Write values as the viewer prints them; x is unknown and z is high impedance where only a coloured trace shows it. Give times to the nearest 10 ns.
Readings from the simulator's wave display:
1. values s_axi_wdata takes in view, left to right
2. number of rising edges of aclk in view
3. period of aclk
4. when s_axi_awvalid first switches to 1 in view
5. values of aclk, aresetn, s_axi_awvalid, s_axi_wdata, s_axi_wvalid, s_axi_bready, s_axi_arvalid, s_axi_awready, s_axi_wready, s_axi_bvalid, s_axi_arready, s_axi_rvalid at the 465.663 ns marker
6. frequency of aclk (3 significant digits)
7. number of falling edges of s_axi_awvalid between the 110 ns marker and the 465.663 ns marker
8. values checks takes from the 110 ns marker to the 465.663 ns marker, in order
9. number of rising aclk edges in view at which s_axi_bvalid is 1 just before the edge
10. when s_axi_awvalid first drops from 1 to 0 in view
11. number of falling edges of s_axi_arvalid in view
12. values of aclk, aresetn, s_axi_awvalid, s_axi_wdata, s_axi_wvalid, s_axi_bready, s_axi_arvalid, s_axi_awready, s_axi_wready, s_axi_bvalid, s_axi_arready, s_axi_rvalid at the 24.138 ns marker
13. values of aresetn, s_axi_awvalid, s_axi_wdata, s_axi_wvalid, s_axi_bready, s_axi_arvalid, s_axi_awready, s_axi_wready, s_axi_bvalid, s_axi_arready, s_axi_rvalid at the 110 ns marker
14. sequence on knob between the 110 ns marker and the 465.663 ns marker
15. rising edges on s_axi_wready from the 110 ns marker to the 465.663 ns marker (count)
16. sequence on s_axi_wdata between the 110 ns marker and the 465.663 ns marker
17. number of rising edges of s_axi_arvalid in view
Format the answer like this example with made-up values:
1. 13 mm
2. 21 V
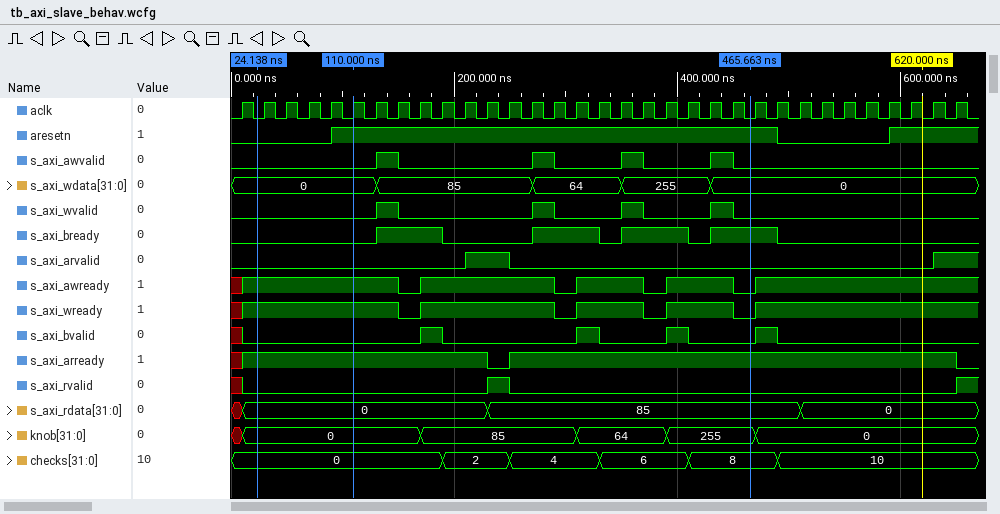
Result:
1. 0, 85, 64, 255, 0
2. 33
3. 20 ns
4. 130 ns
5. aclk=0, aresetn=1, s_axi_awvalid=0, s_axi_wdata=0, s_axi_wvalid=0, s_axi_bready=1, s_axi_arvalid=0, s_axi_awready=0, s_axi_wready=0, s_axi_bvalid=0, s_axi_arready=1, s_axi_rvalid=0
6. 50.0 MHz
7. 4
8. 0, 2, 4, 6, 8
9. 4
10. 150 ns
11. 1
12. aclk=0, aresetn=0, s_axi_awvalid=0, s_axi_wdata=0, s_axi_wvalid=0, s_axi_bready=0, s_axi_arvalid=0, s_axi_awready=1, s_axi_wready=1, s_axi_bvalid=0, s_axi_arready=1, s_axi_rvalid=0
13. aresetn=1, s_axi_awvalid=0, s_axi_wdata=0, s_axi_wvalid=0, s_axi_bready=0, s_axi_arvalid=0, s_axi_awready=1, s_axi_wready=1, s_axi_bvalid=0, s_axi_arready=1, s_axi_rvalid=0
14. 0, 85, 64, 255
15. 3
16. 0, 85, 64, 255, 0
17. 2
